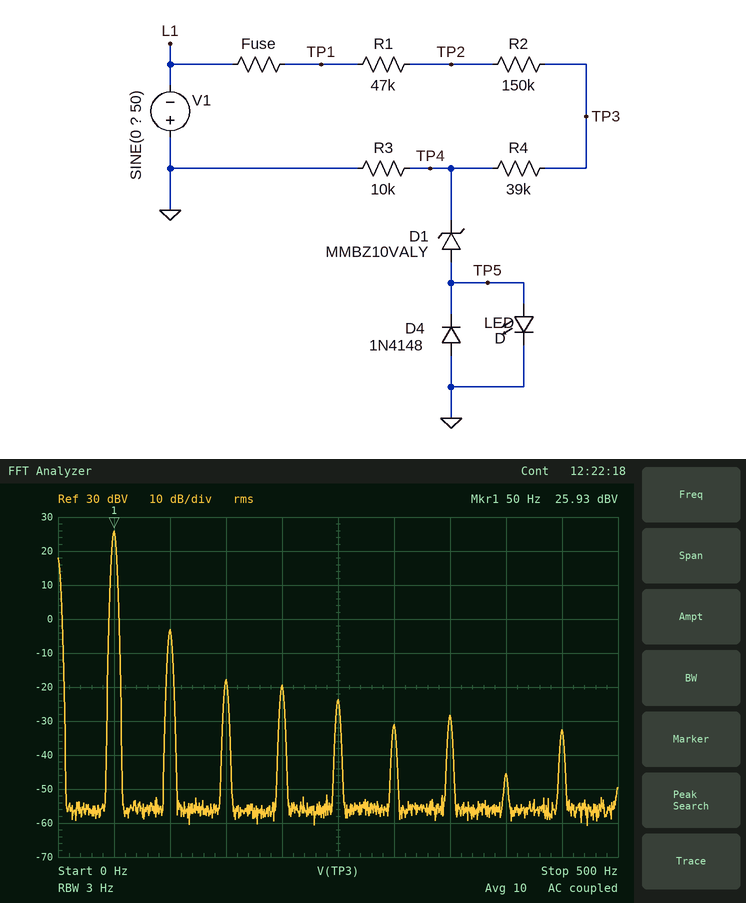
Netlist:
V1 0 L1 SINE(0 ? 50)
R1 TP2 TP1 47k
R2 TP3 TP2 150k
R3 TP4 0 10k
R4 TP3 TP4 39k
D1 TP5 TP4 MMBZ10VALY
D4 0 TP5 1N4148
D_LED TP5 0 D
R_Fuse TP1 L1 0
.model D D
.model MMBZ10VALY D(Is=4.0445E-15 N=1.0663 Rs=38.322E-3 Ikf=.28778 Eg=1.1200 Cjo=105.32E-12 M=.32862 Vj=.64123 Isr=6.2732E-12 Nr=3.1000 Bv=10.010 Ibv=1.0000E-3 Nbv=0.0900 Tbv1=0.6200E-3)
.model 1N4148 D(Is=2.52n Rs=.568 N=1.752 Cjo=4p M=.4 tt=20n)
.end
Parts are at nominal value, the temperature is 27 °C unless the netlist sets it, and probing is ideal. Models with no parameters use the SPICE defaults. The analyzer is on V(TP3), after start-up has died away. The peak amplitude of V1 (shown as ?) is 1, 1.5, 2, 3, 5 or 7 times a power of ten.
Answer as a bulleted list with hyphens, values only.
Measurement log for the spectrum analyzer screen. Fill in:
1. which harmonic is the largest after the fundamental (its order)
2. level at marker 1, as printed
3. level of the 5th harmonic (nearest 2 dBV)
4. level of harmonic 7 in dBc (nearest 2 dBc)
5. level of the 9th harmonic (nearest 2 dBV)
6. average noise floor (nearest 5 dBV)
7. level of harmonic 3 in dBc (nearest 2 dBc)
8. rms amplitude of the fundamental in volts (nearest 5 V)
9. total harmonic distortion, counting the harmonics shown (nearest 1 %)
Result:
- 2
- 25.93 dBV
- -24 dBV
- -54 dBc
- -32 dBV
- -55 dBV
- -44 dBc
- 20 V
- 4 %
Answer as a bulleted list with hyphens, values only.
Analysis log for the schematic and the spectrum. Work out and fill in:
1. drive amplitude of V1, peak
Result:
- 150 V
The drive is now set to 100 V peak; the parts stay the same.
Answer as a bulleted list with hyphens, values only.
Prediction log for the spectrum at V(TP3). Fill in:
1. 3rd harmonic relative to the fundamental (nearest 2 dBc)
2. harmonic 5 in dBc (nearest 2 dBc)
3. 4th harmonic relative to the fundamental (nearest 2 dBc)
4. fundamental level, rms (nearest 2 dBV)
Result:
- -42 dBc
- -48 dBc
- -50 dBc
- 22 dBV
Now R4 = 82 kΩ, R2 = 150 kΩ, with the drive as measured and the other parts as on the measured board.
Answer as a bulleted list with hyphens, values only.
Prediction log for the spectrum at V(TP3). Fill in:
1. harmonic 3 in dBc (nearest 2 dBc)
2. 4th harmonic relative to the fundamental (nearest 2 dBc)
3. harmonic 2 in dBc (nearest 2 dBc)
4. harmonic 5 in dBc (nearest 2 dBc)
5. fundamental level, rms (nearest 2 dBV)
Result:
- -50 dBc
- -54 dBc
- -36 dBc
- -56 dBc
- 30 dBV
